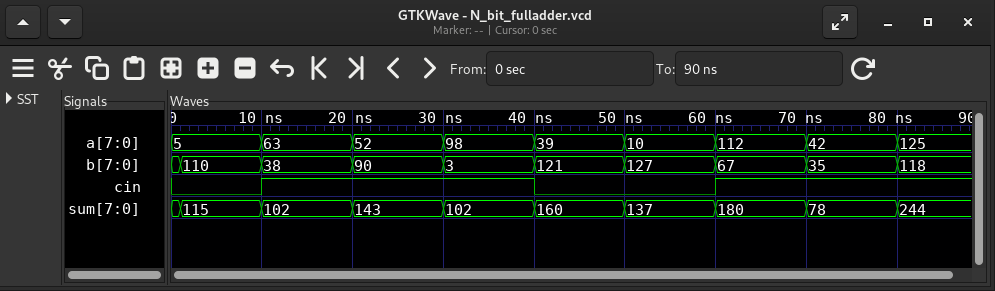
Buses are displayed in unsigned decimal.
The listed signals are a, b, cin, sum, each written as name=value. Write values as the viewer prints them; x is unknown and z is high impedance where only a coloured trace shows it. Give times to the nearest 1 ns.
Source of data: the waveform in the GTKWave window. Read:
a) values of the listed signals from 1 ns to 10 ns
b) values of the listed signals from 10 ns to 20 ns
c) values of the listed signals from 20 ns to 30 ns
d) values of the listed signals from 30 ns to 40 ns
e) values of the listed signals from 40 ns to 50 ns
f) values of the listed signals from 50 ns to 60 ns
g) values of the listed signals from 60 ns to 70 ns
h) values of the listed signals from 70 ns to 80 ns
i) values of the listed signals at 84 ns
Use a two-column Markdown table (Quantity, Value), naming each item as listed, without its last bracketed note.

| Quantity | Value |
|---|---|
| values of the listed signals from 1 ns to 10 ns | a=5, b=110, cin=0, sum=115 |
| values of the listed signals from 10 ns to 20 ns | a=63, b=38, cin=1, sum=102 |
| values of the listed signals from 20 ns to 30 ns | a=52, b=90, cin=1, sum=143 |
| values of the listed signals from 30 ns to 40 ns | a=98, b=3, cin=1, sum=102 |
| values of the listed signals from 40 ns to 50 ns | a=39, b=121, cin=0, sum=160 |
| values of the listed signals from 50 ns to 60 ns | a=10, b=127, cin=0, sum=137 |
| values of the listed signals from 60 ns to 70 ns | a=112, b=67, cin=1, sum=180 |
| values of the listed signals from 70 ns to 80 ns | a=42, b=35, cin=1, sum=78 |
| values of the listed signals at 84 ns | a=125, b=118, cin=1, sum=244 |
